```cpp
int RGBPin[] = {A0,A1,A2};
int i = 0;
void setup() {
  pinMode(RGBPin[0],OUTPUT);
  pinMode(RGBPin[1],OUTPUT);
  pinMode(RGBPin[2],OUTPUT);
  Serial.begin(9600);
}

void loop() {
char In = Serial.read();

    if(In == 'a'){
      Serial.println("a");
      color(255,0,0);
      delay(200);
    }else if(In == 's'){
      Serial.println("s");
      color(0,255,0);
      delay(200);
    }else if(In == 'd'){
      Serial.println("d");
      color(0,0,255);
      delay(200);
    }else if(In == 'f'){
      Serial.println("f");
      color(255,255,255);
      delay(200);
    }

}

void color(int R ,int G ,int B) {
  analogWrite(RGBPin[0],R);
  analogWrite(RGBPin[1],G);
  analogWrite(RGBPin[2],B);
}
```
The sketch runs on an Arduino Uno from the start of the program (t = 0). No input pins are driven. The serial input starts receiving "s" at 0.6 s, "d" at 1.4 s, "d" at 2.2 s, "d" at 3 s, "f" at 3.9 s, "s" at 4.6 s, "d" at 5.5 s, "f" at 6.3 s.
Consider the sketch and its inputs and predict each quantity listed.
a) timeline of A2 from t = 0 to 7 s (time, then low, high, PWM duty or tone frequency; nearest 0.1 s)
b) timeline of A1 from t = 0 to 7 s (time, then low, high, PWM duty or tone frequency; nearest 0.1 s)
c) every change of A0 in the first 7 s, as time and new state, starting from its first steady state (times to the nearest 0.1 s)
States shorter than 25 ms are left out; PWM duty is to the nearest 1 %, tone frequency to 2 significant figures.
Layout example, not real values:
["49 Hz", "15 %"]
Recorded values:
["0 s low; 1.4 s high; 4.6 s low; 5.5 s high", "0 s low; 0.6 s high; 1.4 s low; 3.9 s high; 5.5 s low; 6.3 s high", "0 s low; 3.9 s high; 4.6 s low; 6.3 s high"]
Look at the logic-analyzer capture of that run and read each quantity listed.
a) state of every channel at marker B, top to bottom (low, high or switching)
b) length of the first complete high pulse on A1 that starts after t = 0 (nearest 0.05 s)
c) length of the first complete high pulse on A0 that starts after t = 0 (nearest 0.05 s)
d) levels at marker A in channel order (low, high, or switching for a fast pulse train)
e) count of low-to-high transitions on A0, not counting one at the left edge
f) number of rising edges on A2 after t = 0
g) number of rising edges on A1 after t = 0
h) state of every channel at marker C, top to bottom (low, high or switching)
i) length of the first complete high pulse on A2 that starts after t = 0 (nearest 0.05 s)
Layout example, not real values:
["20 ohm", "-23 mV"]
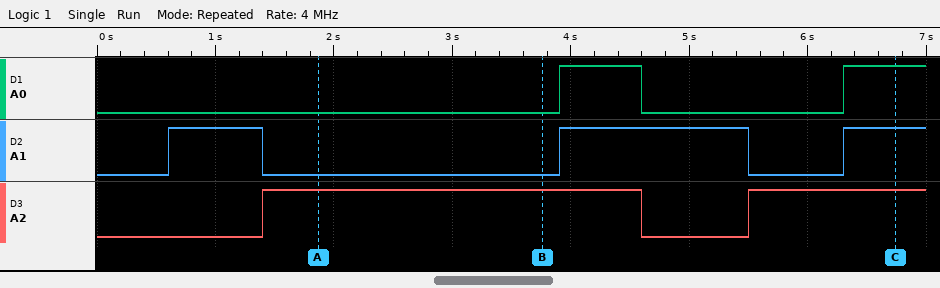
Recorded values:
["A0 low, A1 low, A2 high", "0.80 s", "0.70 s", "A0 low, A1 low, A2 high", "2", "2", "3", "A0 high, A1 high, A2 high", "3.20 s"]
